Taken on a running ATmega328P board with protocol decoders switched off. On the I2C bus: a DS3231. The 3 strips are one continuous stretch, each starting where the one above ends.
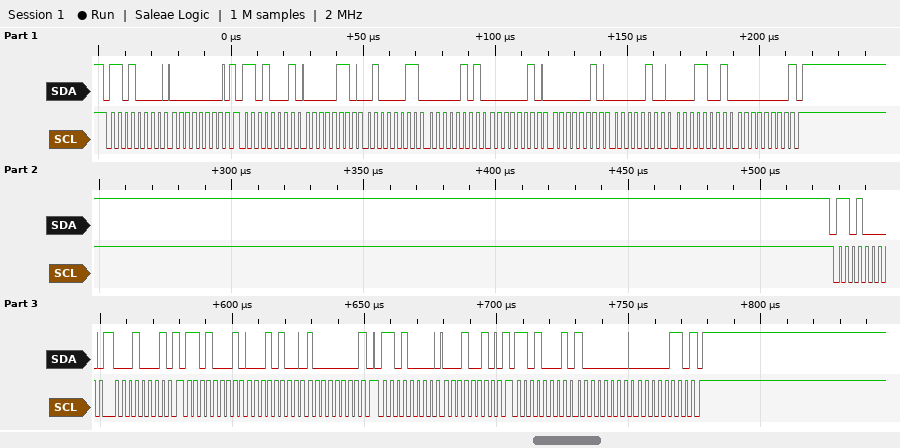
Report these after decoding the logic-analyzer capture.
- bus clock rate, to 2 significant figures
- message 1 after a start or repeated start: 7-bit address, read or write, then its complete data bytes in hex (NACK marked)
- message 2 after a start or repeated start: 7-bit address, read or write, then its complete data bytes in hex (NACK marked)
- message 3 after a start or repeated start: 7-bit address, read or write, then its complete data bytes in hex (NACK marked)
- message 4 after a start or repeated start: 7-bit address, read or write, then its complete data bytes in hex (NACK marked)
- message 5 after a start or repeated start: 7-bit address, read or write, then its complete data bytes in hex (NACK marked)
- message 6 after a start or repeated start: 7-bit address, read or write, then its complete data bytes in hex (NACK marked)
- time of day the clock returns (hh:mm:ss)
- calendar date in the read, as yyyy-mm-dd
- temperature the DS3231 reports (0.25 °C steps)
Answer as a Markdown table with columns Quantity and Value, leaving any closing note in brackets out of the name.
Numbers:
| Quantity | Value |
|---|---|
| bus clock rate, to 2 significant figures | 400 kHz |
| message 1 after a start or repeated start: 7-bit address, read or write, then its complete data bytes in hex | 0x68 write: 00 |
| message 2 after a start or repeated start: 7-bit address, read or write, then its complete data bytes in hex | 0x68 read: 06 43 05 02 02 04 19 00 NACK |
| message 3 after a start or repeated start: 7-bit address, read or write, then its complete data bytes in hex | 0x68 write: 11 |
| message 4 after a start or repeated start: 7-bit address, read or write, then its complete data bytes in hex | 0x68 read: 14 80 NACK |
| message 5 after a start or repeated start: 7-bit address, read or write, then its complete data bytes in hex | 0x68 write: 12 |
| message 6 after a start or repeated start: 7-bit address, read or write, then its complete data bytes in hex | 0x68 read: 80 06 NACK |
| time of day the clock returns | 05:43:06 |
| calendar date in the read, as yyyy-mm-dd | 2019-04-02 |
| temperature the DS3231 reports | 20.50 °C |
